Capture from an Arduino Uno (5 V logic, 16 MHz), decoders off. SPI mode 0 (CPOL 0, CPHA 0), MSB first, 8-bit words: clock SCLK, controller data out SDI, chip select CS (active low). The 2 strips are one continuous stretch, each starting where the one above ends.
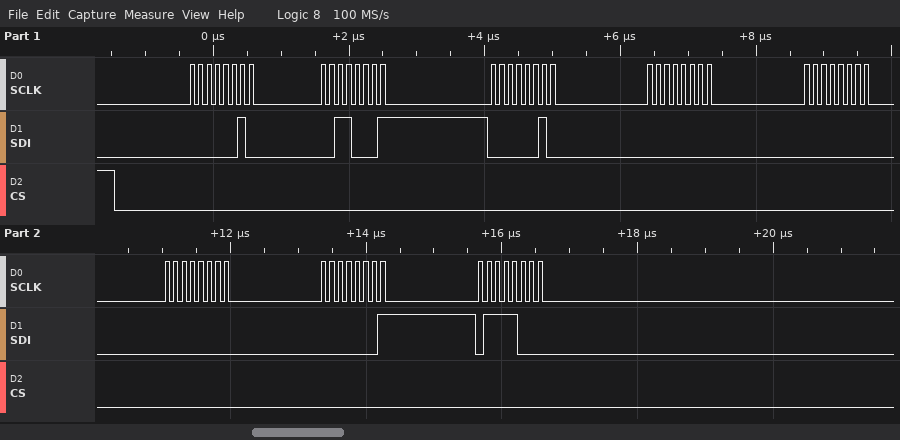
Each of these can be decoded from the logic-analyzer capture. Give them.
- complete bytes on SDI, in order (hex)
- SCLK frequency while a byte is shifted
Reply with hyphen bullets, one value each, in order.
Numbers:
- 02 31 02 00 00 00 01 78
- 8 MHz
